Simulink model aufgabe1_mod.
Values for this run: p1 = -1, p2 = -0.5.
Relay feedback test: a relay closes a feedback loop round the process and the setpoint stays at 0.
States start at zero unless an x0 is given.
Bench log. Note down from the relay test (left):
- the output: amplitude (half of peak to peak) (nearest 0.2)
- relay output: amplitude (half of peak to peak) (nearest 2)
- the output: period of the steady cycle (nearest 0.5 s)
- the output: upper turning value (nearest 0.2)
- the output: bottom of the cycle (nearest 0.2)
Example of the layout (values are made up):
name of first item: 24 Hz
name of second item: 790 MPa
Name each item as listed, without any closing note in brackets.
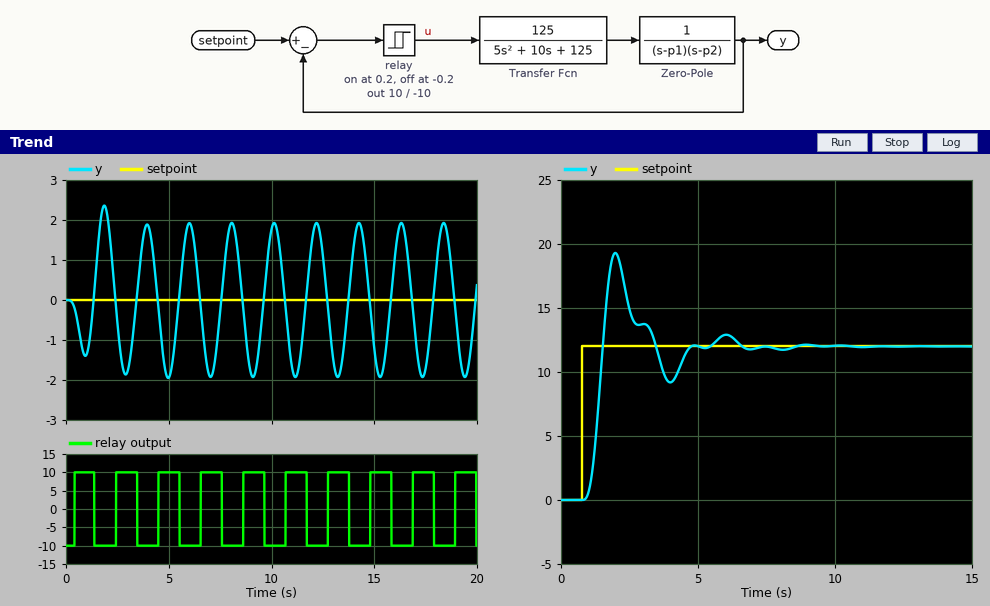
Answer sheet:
the output: amplitude (half of peak to peak): 2.0
relay output: amplitude (half of peak to peak): 10
the output: period of the steady cycle: 2.0 s
the output: upper turning value: 2.0
the output: bottom of the cycle: -2.0
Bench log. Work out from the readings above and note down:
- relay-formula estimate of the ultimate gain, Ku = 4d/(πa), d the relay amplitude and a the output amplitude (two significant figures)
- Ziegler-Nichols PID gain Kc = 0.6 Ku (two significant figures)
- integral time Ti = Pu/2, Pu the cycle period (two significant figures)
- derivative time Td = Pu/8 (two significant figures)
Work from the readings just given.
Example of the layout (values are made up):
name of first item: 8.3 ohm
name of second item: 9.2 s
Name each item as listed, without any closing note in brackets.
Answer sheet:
relay-formula estimate of the ultimate gain, Ku = 4d/(πa), d the relay amplitude and a the output amplitude: 6.4
Ziegler-Nichols PID gain Kc = 0.6 Ku: 3.8
integral time Ti = Pu/2, Pu the cycle period: 1.0 s
derivative time Td = Pu/8: 0.25 s
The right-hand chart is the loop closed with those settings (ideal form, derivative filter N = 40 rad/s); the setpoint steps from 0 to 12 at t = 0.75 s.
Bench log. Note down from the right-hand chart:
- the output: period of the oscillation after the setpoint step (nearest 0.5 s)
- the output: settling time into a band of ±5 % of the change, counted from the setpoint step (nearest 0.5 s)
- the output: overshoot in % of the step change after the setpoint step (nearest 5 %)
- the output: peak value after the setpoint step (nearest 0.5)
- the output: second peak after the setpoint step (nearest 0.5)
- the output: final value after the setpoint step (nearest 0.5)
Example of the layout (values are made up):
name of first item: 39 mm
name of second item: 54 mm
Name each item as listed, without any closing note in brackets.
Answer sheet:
the output: period of the oscillation after the setpoint step: 4.0 s
the output: settling time into a band of ±5 % of the change, counted from the setpoint step: 5.5 s
the output: overshoot in % of the step change after the setpoint step: 60 %
the output: peak value after the setpoint step: 19.5
the output: second peak after the setpoint step: 13.0
the output: final value after the setpoint step: 12.0
